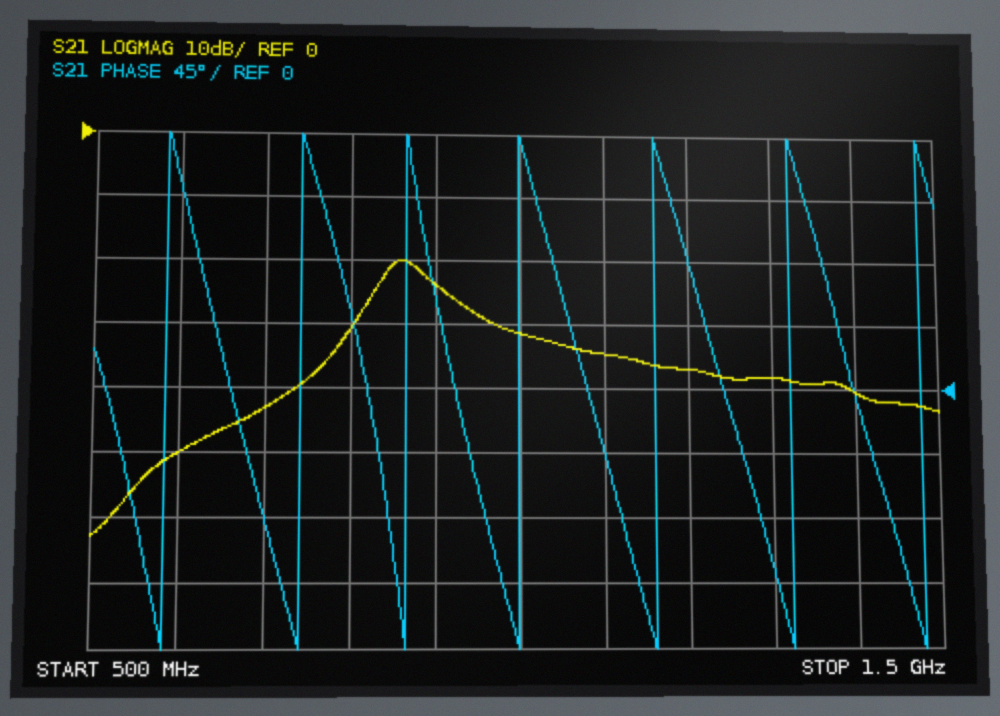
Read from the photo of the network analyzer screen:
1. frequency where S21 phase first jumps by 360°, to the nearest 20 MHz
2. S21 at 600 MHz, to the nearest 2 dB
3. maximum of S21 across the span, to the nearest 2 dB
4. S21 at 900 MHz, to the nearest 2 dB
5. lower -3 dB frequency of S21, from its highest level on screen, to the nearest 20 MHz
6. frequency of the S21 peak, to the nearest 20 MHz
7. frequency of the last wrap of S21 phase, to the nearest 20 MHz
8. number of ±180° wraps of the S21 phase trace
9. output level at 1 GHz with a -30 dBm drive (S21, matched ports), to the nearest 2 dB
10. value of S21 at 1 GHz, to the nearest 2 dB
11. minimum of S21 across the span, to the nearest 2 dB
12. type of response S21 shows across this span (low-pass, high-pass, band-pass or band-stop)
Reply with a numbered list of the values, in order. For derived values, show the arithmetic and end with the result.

1. 580 MHz
2. -50 dB
3. -20 dB
4. -24 dB
5. 840 MHz
6. 860 MHz
7. 1.48 GHz
8. 7
9. -30 dBm + (-32 dB) = -62 dBm
10. -32 dB
11. -62 dB
12. band-pass
